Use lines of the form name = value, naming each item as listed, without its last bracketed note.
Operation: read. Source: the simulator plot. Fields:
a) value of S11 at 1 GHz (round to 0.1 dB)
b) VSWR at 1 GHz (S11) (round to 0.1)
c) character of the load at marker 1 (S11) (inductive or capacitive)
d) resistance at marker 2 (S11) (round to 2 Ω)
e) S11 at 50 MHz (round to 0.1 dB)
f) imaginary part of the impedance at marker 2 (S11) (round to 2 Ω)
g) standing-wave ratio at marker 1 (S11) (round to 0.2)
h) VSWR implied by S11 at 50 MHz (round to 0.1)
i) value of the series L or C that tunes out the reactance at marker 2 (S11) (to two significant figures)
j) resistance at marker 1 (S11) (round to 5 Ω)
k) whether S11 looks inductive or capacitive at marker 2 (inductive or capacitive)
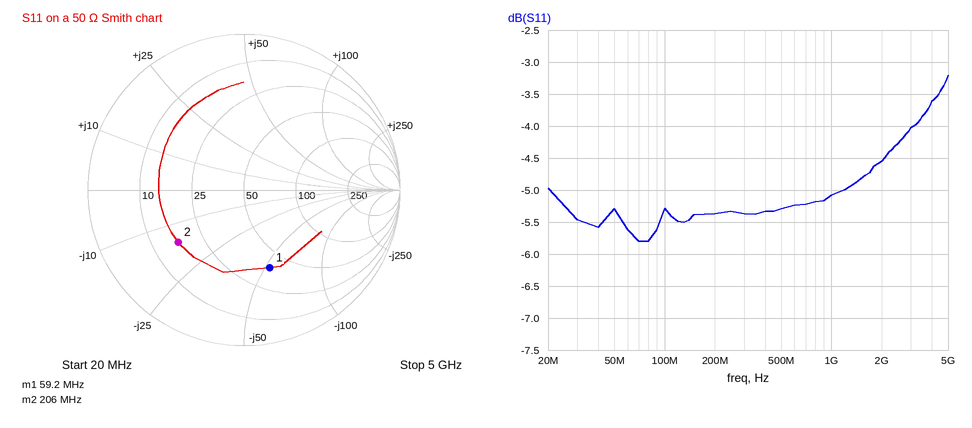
value of S11 at 1 GHz = -5.1 dB
VSWR at 1 GHz (S11) = 3.5
character of the load at marker 1 (S11) = capacitive
resistance at marker 2 (S11) = 16 Ω
S11 at 50 MHz = -5.3 dB
imaginary part of the impedance at marker 2 (S11) = -16 Ω
standing-wave ratio at marker 1 (S11) = 3.2
VSWR implied by S11 at 50 MHz = 3.4
value of the series L or C that tunes out the reactance at marker 2 (S11) = 12 nH
resistance at marker 1 (S11) = 40 Ω
whether S11 looks inductive or capacitive at marker 2 = capacitive
